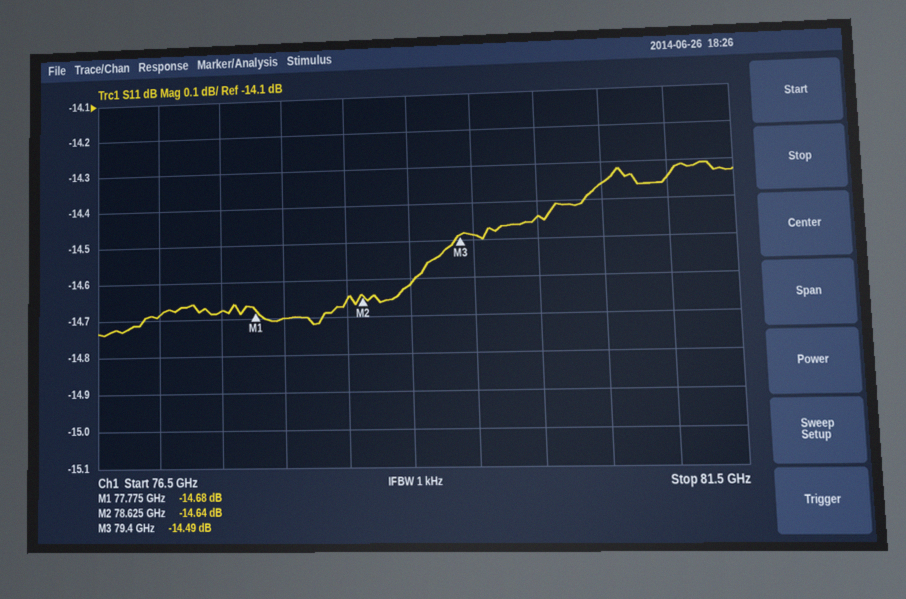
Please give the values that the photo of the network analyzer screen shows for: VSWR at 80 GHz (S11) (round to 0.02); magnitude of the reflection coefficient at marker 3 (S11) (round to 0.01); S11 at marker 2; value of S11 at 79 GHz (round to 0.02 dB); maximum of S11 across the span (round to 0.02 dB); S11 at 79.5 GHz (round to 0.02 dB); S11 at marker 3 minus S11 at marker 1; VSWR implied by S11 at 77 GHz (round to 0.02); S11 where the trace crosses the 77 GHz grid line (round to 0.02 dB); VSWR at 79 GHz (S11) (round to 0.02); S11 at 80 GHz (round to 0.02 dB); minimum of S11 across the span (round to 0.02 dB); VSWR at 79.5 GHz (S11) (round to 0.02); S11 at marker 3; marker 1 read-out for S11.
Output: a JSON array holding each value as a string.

["1.46", "0.19", "-14.64 dB", "-14.62 dB", "-14.30 dB", "-14.48 dB", "0.19 dB", "1.46", "-14.68 dB", "1.46", "-14.44 dB", "-14.74 dB", "1.46", "-14.49 dB", "-14.68 dB"]
